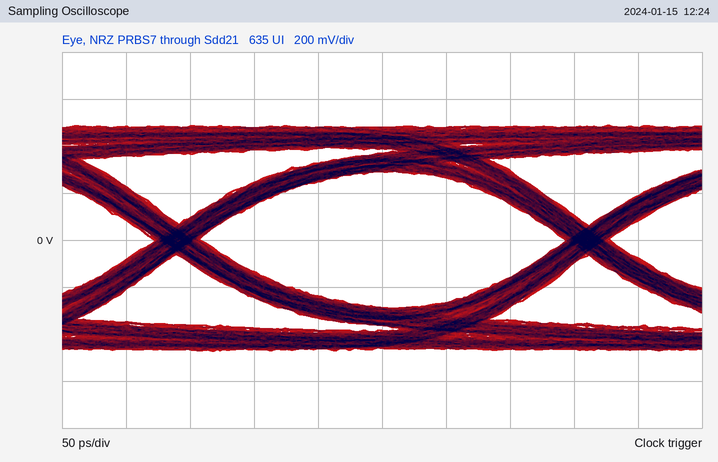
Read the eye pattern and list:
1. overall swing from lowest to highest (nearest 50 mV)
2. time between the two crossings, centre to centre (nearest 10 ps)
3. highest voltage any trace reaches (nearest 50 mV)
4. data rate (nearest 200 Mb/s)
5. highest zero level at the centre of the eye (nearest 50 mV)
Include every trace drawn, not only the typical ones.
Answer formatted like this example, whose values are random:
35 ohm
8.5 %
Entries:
950 mV
320 ps
500 mV
3.2 Gb/s
-300 mV
